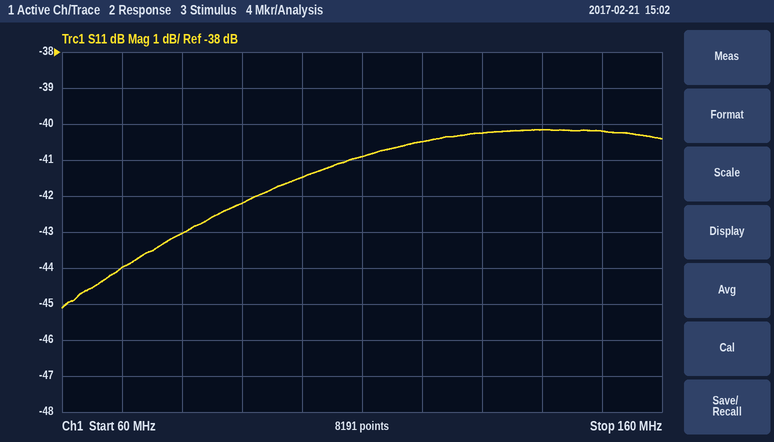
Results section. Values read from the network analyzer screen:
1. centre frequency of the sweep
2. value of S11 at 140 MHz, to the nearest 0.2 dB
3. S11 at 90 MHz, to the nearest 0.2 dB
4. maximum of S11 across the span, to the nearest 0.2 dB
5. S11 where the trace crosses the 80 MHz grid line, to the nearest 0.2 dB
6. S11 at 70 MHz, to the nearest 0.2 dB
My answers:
110 MHz
-40.2 dB
-42.2 dB
-40.2 dB
-43.0 dB
-44.0 dB
